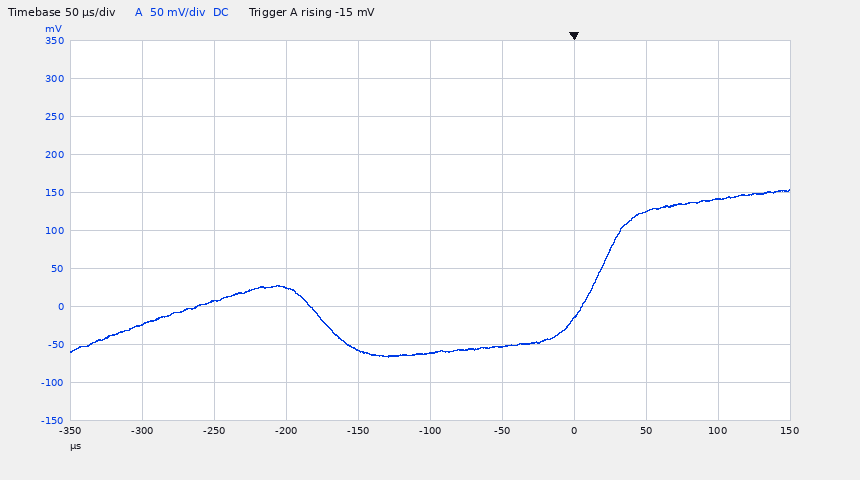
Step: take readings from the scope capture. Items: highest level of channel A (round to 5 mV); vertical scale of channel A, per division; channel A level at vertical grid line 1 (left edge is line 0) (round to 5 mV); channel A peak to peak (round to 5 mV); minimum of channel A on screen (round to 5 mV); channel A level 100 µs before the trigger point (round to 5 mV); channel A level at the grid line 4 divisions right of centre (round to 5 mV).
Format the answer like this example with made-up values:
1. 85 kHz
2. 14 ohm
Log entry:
1. 155 mV
2. 50 mV
3. -25 mV
4. 220 mV
5. -65 mV
6. -60 mV
7. 140 mV
